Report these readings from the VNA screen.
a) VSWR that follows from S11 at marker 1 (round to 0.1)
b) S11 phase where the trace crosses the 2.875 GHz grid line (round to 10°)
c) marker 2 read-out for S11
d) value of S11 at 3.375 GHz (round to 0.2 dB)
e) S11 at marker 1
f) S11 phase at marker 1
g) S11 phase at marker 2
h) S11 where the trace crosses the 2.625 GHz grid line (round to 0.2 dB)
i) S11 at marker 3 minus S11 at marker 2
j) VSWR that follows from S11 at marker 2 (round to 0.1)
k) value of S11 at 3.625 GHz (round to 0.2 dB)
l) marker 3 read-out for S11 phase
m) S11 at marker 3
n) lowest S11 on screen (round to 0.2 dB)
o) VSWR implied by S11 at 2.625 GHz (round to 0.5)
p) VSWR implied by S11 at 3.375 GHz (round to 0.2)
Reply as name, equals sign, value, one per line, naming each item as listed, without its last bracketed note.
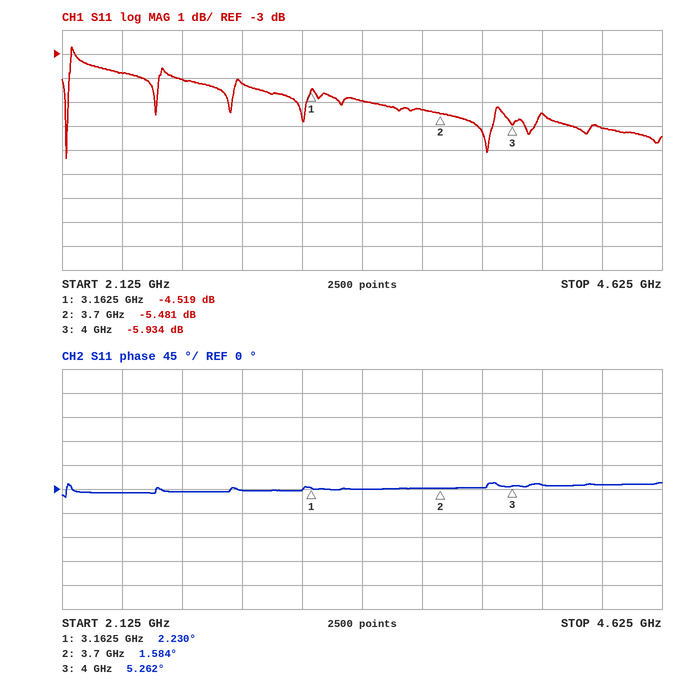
VSWR that follows from S11 at marker 1 = 3.9
S11 phase where the trace crosses the 2.875 GHz grid line = 0°
marker 2 read-out for S11 = -5.481 dB
value of S11 at 3.375 GHz = -5.0 dB
S11 at marker 1 = -4.519 dB
S11 phase at marker 1 = 2.230°
S11 phase at marker 2 = 1.584°
S11 where the trace crosses the 2.625 GHz grid line = -4.0 dB
S11 at marker 3 minus S11 at marker 2 = -0.453 dB
VSWR that follows from S11 at marker 2 = 3.3
value of S11 at 3.625 GHz = -5.4 dB
marker 3 read-out for S11 phase = 5.262°
S11 at marker 3 = -5.934 dB
lowest S11 on screen = -7.4 dB
VSWR implied by S11 at 2.625 GHz = 4.5
VSWR implied by S11 at 3.375 GHz = 3.6
